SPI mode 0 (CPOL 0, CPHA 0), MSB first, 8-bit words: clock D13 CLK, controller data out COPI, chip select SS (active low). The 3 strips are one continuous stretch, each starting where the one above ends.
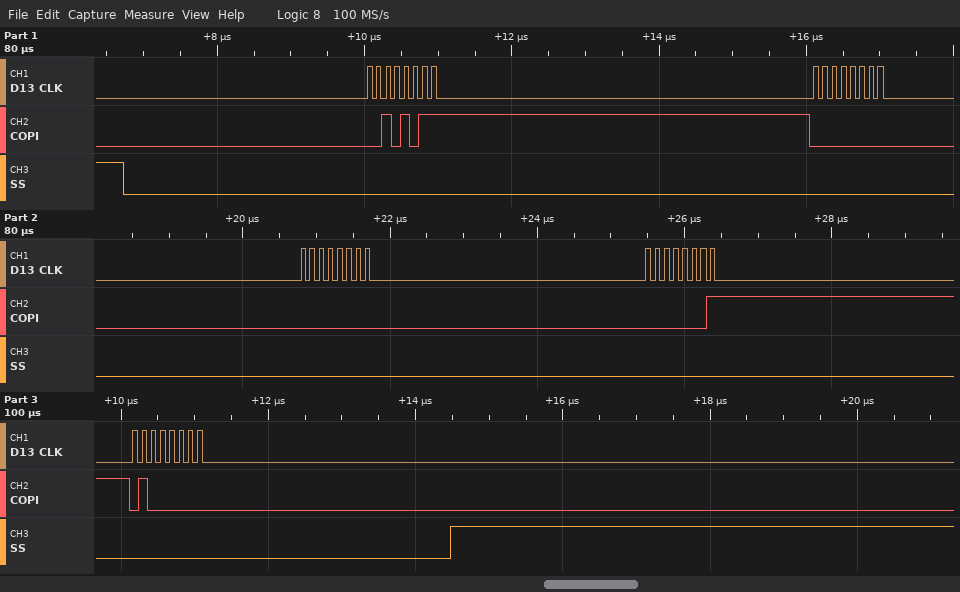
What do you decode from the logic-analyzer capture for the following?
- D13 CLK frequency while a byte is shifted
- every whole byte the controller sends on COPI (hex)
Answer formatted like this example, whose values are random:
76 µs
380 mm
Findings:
8 MHz
2B 00 00 01 40
